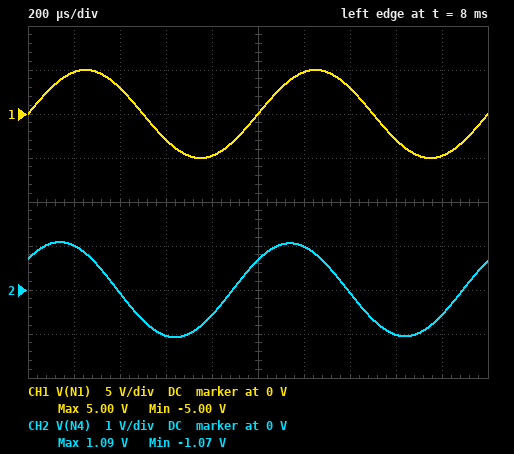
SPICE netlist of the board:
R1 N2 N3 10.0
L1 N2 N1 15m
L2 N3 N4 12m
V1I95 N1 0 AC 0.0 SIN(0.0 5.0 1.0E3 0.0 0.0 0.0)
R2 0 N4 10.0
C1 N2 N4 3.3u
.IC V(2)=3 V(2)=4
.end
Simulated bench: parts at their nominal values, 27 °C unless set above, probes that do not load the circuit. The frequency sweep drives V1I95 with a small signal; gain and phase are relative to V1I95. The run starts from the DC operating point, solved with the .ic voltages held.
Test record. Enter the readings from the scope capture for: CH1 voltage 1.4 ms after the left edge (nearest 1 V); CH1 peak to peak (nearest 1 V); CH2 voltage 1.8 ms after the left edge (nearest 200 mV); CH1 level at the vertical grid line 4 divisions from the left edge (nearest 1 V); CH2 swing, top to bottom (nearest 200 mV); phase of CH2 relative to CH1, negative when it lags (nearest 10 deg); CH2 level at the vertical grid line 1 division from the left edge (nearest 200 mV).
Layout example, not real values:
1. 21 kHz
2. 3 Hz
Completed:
1. 3 V
2. 10 V
3. -600 mV
4. -5 V
5. 2.2 V
6. 40 deg
7. 1.0 V
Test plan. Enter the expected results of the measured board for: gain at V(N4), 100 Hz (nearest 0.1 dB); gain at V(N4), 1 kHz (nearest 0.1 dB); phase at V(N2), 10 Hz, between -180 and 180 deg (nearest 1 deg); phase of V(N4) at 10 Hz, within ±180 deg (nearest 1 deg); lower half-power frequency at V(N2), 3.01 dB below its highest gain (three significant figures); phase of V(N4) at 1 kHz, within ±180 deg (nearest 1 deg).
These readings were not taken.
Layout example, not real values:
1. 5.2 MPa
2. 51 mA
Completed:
1. -8.4 dB
2. -13.6 dB
3. -3 deg
4. -5 deg
5. 1.01 kHz
6. 38 deg
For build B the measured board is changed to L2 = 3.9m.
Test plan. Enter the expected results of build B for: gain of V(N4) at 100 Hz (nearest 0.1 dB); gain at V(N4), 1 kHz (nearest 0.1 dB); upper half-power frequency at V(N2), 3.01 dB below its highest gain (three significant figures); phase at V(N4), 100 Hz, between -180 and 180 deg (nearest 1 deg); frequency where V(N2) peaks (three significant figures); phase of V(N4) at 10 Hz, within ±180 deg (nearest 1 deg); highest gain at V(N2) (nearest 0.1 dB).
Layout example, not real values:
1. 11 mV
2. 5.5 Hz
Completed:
1. -7.3 dB
2. -22.7 dB
3. 1.71 kHz
4. -30 deg
5. 1.55 kHz
6. -3 deg
7. 0.4 dB
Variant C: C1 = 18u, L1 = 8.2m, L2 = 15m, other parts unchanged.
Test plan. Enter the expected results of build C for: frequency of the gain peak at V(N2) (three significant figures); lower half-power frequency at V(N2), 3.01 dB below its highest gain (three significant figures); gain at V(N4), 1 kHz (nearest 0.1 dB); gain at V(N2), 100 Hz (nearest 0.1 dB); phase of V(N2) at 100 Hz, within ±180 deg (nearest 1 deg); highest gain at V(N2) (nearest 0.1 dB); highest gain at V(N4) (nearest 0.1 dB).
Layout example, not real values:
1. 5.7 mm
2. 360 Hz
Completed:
1. 503 Hz
2. 415 Hz
3. -12.7 dB
4. -0.8 dB
5. -10 deg
6. 7.1 dB
7. -2.0 dB
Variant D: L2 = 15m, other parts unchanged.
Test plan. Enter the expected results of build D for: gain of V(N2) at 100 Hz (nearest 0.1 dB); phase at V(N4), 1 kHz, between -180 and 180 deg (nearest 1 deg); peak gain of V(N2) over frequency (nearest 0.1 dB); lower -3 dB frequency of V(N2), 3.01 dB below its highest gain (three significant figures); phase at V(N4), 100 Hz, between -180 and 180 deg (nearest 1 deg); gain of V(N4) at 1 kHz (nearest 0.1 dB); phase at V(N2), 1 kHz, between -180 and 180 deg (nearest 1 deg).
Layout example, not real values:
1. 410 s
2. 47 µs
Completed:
1. -1.8 dB
2. 6 deg
3. 13.7 dB
4. 954 Hz
5. -43 deg
6. -6.3 dB
7. -72 deg
